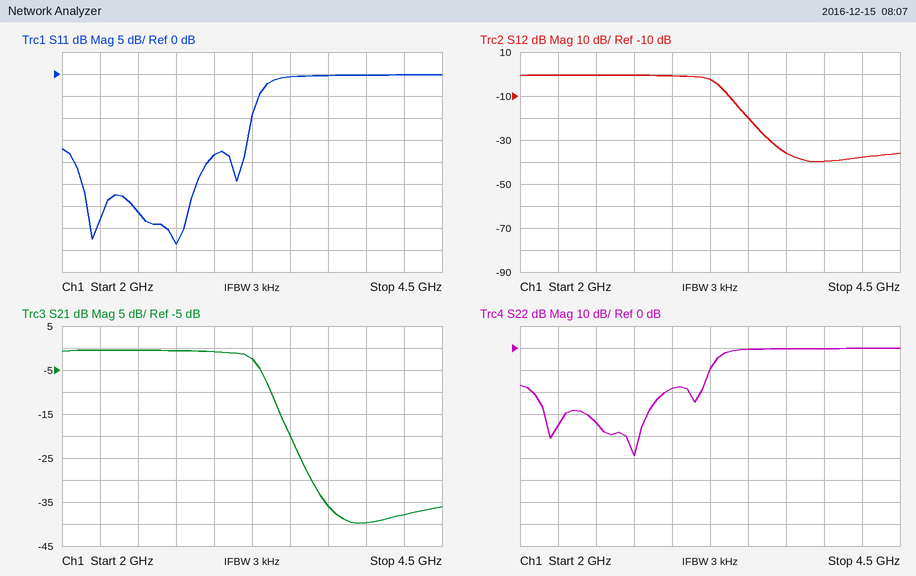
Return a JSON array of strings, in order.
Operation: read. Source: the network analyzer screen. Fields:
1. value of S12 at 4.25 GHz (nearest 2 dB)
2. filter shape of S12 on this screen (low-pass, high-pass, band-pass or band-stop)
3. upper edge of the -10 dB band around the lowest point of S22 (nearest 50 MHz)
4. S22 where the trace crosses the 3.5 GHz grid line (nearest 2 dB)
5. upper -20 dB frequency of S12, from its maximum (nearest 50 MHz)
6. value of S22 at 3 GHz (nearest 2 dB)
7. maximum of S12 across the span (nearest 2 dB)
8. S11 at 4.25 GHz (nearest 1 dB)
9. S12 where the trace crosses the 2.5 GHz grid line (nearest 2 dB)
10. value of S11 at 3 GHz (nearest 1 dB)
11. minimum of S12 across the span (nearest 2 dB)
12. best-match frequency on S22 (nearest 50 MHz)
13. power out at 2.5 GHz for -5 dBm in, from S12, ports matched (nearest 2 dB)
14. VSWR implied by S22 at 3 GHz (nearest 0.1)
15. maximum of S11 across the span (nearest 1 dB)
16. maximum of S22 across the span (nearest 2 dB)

["-38 dB", "low-pass", "3.25 GHz", "0 dB", "3.50 GHz", "-18 dB", "0 dB", "0 dB", "0 dB", "-18 dB", "-40 dB", "2.75 GHz", "-6 dBm", "1.3", "0 dB", "0 dB"]
